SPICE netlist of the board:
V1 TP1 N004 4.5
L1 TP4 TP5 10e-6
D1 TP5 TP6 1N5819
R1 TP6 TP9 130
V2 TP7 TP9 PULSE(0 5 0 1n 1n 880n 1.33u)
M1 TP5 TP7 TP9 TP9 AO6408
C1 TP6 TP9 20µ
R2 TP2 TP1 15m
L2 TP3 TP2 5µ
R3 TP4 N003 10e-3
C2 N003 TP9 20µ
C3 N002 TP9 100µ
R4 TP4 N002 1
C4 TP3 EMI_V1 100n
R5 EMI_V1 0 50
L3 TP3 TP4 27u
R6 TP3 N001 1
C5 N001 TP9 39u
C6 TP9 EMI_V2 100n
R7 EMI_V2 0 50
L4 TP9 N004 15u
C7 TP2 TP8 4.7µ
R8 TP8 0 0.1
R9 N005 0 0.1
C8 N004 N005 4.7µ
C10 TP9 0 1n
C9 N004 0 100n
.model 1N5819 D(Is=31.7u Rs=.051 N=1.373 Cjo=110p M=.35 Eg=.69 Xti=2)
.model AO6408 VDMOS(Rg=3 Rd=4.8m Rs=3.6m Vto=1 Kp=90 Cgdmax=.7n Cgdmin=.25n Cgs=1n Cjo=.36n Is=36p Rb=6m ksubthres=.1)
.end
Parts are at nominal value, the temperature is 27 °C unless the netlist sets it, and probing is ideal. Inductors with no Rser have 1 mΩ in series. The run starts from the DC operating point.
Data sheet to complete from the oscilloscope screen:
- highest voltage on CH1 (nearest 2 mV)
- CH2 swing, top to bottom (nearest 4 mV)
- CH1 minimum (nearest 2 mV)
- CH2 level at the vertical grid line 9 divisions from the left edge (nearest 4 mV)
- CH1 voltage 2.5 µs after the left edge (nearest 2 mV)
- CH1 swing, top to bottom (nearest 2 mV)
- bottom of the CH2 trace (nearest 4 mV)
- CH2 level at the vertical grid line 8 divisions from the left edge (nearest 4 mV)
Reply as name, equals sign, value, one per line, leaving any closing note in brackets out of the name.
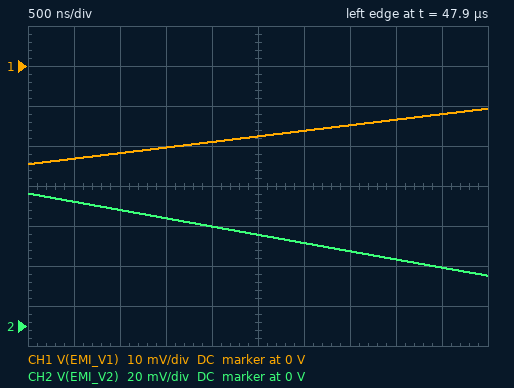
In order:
highest voltage on CH1 = -10 mV
CH2 swing, top to bottom = 40 mV
CH1 minimum = -24 mV
CH2 level at the vertical grid line 9 divisions from the left edge = 28 mV
CH1 voltage 2.5 µs after the left edge = -18 mV
CH1 swing, top to bottom = 14 mV
bottom of the CH2 trace = 24 mV
CH2 level at the vertical grid line 8 divisions from the left edge = 32 mV
